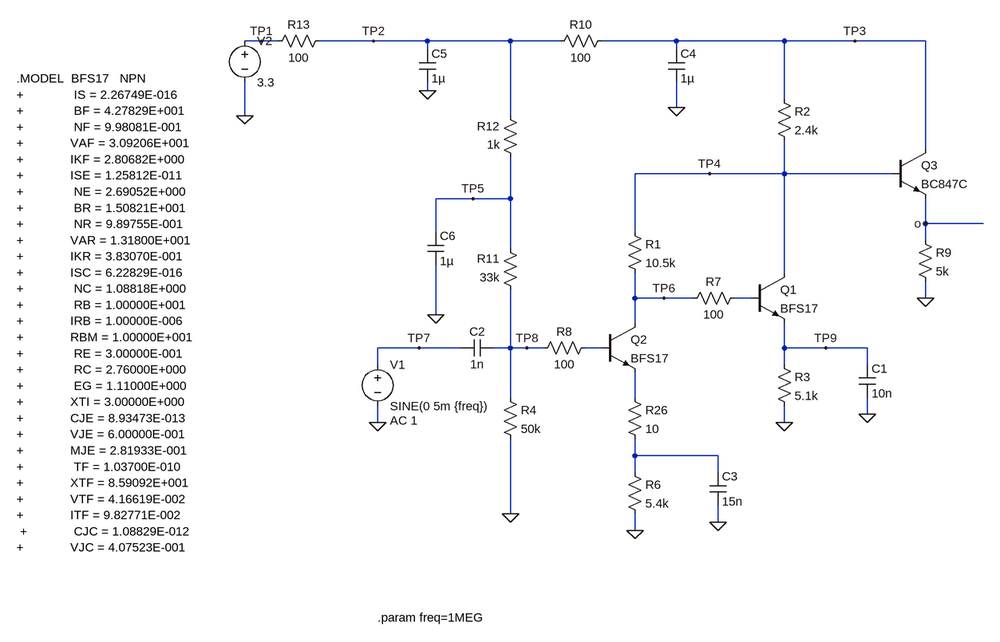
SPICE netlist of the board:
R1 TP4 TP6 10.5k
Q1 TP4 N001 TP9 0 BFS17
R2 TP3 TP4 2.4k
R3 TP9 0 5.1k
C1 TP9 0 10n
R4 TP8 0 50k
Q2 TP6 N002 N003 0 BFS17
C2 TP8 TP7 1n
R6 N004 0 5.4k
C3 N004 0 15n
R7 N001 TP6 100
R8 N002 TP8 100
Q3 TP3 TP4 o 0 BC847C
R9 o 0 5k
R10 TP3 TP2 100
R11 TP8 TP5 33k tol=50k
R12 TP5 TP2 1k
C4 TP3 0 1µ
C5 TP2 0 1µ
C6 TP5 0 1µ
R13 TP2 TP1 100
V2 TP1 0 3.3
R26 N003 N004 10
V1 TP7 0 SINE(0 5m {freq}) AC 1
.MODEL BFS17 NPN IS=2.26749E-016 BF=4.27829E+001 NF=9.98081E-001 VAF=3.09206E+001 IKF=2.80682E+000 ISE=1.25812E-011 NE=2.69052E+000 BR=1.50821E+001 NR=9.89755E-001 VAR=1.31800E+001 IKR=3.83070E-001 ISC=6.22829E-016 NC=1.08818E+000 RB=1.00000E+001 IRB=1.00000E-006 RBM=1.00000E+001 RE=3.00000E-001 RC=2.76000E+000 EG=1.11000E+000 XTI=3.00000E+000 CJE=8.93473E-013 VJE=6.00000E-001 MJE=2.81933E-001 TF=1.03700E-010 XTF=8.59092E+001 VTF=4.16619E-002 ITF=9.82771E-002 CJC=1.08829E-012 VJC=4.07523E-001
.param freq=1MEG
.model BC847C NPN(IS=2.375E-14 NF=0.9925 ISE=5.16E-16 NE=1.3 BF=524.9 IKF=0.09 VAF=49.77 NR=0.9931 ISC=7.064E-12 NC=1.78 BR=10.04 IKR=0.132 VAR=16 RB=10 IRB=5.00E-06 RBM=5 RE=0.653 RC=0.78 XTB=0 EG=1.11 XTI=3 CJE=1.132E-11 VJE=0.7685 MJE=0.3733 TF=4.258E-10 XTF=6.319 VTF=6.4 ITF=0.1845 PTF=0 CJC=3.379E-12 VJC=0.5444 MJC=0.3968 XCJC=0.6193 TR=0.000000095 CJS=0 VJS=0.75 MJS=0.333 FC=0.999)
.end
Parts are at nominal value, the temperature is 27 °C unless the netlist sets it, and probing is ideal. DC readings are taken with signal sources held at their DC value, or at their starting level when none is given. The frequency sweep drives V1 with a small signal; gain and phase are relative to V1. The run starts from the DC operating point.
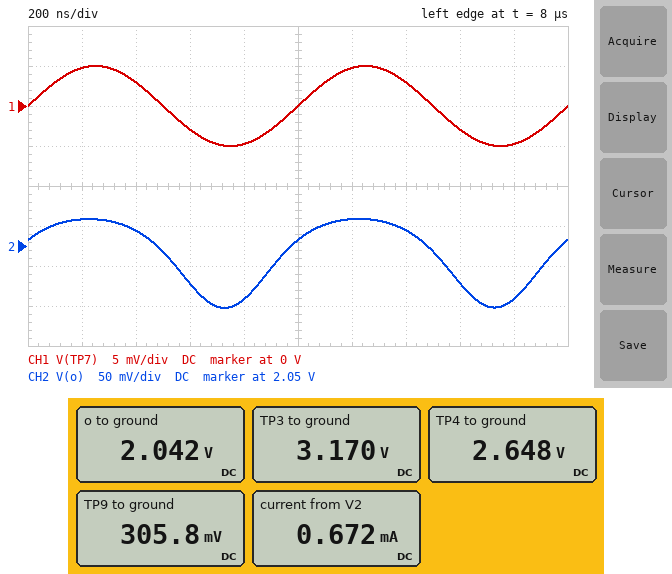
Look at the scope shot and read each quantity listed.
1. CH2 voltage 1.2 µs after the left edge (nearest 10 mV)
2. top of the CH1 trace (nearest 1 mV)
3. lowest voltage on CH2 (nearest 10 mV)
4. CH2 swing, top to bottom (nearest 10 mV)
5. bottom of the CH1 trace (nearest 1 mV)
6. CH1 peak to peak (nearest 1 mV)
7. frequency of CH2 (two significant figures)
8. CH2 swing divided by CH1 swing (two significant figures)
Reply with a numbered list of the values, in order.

1. 2.08 V
2. 5 mV
3. 1.97 V
4. 110 mV
5. -5 mV
6. 10 mV
7. 1.0 MHz
8. 11
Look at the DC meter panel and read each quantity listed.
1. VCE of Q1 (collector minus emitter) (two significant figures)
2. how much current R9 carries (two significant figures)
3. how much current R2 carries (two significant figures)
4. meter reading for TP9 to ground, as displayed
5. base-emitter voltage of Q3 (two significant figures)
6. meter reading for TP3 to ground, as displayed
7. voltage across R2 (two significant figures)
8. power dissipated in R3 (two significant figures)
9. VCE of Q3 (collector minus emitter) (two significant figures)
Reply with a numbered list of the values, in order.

1. 2.3 V
2. 410 µA
3. 220 µA
4. 305.8 mV
5. 610 mV
6. 3.170 V
7. 520 mV
8. 18 µW
9. 1.1 V
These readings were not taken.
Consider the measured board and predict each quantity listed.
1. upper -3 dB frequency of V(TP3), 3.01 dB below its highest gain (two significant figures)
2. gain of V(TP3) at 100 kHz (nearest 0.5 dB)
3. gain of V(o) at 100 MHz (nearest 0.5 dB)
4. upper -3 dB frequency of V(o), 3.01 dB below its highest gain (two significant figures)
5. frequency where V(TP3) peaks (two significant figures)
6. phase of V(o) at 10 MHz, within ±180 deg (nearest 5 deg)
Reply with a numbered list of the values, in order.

1. 300 kHz
2. -57.0 dB
3. -9.0 dB
4. 13 MHz
5. 95 kHz
6. -60 deg
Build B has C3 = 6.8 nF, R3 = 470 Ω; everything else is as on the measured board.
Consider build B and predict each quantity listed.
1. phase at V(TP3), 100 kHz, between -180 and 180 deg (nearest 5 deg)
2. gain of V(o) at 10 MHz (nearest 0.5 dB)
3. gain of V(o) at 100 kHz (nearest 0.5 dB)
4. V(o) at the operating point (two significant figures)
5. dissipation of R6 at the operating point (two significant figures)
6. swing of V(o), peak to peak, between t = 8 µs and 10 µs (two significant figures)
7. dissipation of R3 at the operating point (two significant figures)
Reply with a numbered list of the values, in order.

1. 35 deg
2. 22.0 dB
3. 11.0 dB
4. 1.6 V
5. 120 µW
6. 150 mV
7. 31 µW
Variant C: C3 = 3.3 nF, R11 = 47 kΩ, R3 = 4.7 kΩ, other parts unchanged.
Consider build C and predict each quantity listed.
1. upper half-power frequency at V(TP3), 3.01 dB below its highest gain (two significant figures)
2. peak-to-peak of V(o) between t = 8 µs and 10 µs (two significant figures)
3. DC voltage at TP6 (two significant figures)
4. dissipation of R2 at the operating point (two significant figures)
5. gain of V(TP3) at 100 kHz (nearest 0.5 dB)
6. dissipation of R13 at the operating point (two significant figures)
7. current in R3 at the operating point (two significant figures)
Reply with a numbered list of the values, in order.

1. 310 kHz
2. 310 mV
3. 1.0 V
4. 120 µW
5. -47.0 dB
6. 44 µW
7. 72 µA
